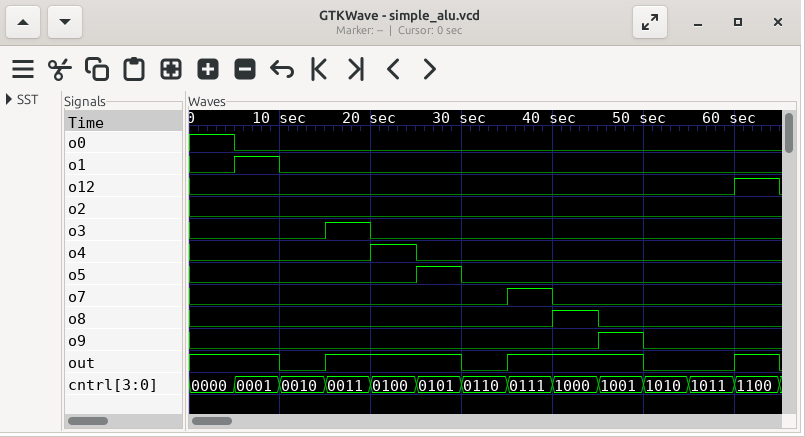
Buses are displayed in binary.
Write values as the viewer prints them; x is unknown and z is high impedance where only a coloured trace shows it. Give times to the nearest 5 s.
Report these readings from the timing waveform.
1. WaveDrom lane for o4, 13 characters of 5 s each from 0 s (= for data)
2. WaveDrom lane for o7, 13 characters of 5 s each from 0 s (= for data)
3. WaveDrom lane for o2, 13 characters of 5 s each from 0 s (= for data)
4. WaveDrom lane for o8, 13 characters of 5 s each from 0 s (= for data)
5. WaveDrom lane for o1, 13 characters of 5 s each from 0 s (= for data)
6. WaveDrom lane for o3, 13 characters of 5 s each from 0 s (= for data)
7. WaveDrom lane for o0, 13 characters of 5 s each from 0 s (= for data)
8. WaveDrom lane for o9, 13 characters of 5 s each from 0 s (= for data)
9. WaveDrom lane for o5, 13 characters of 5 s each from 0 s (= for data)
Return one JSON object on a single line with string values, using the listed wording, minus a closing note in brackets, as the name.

{"WaveDrom lane for o4, 13 characters of 5 s each from 0 s": "{name: 'o4', wave: '0...10.......'}", "WaveDrom lane for o7, 13 characters of 5 s each from 0 s": "{name: 'o7', wave: '0......10....'}", "WaveDrom lane for o2, 13 characters of 5 s each from 0 s": "{name: 'o2', wave: '0............'}", "WaveDrom lane for o8, 13 characters of 5 s each from 0 s": "{name: 'o8', wave: '0.......10...'}", "WaveDrom lane for o1, 13 characters of 5 s each from 0 s": "{name: 'o1', wave: '010..........'}", "WaveDrom lane for o3, 13 characters of 5 s each from 0 s": "{name: 'o3', wave: '0..10........'}", "WaveDrom lane for o0, 13 characters of 5 s each from 0 s": "{name: 'o0', wave: '10...........'}", "WaveDrom lane for o9, 13 characters of 5 s each from 0 s": "{name: 'o9', wave: '0........10..'}", "WaveDrom lane for o5, 13 characters of 5 s each from 0 s": "{name: 'o5', wave: '0....10......'}"}
